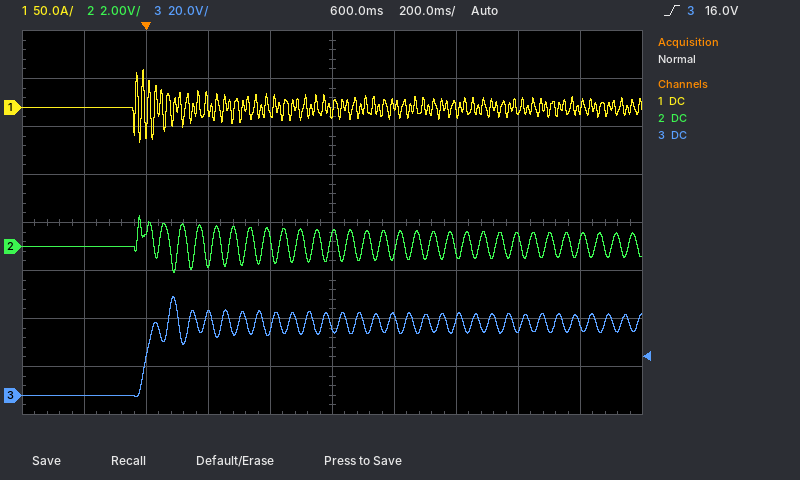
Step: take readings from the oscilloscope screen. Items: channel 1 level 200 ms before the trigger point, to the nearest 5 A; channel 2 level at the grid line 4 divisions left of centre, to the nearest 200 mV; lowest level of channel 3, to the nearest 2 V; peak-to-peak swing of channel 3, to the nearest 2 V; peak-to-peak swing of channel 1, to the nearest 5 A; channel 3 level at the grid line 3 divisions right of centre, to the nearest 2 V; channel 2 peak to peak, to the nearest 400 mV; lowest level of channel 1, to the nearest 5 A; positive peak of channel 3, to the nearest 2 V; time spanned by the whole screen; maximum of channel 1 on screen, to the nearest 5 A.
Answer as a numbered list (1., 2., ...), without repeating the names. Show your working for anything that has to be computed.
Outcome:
1. 0 A
2. 0.0 V
3. 0 V
4. 42 V − (0 V) = 42 V
5. 40 A − (-35 A) = 75 A
6. 28 V
7. 2.4 V
8. -35 A
9. 42 V
10. 2 s
11. 40 A
